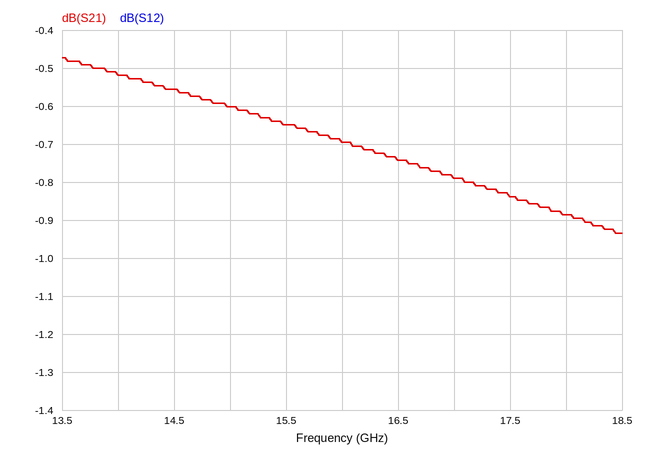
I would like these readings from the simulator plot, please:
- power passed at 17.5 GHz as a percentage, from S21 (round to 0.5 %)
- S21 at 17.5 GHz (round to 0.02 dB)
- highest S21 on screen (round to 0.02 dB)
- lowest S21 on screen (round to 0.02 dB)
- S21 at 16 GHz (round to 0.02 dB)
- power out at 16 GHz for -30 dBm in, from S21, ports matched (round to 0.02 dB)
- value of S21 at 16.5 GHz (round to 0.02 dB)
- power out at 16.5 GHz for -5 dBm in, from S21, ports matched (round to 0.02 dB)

82.5 %
-0.84 dB
-0.48 dB
-0.94 dB
-0.70 dB
-30.70 dBm
-0.74 dB
-5.74 dBm
